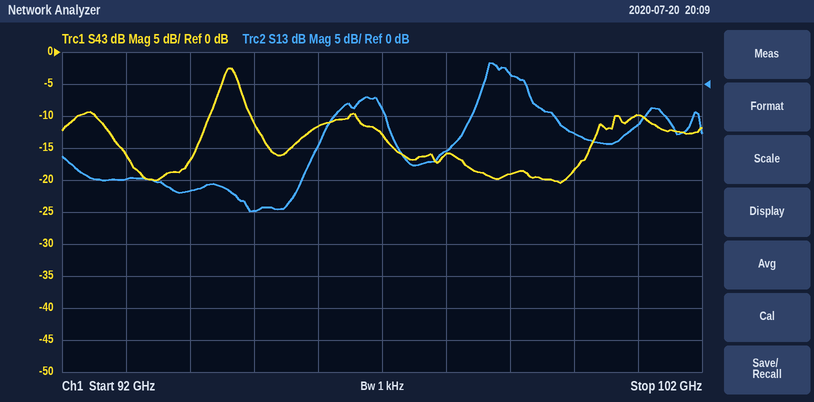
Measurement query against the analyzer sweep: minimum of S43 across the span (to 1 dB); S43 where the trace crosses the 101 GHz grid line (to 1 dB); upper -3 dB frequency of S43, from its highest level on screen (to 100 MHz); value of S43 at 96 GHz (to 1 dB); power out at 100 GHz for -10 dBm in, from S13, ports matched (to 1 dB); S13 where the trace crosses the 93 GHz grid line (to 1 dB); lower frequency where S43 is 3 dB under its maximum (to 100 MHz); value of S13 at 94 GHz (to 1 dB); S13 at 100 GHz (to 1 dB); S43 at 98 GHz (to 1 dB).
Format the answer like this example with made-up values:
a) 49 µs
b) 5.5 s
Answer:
a) -20 dB
b) -10 dB
c) 94.8 GHz
d) -12 dB
e) -18 dBm
f) -15 dB
g) 94.5 GHz
h) -17 dB
i) -8 dB
j) -16 dB
